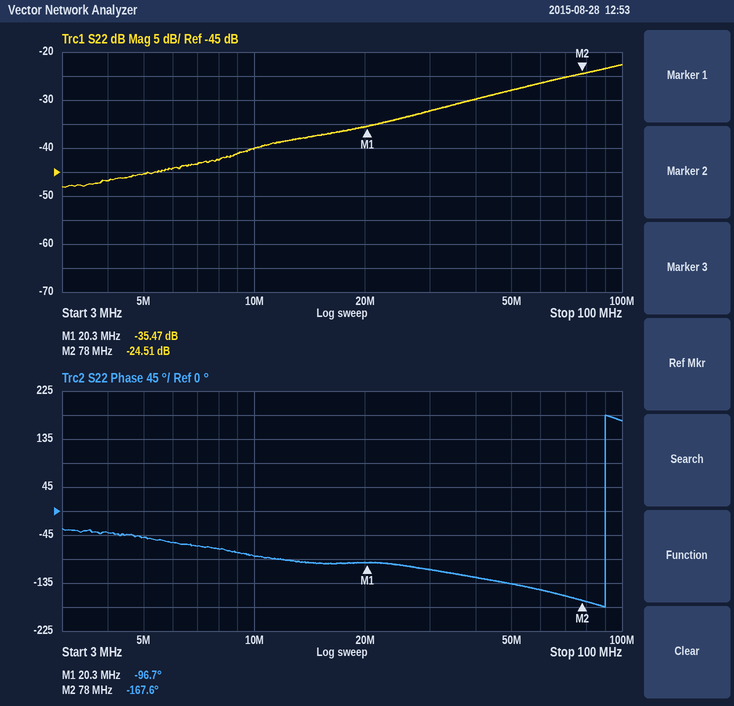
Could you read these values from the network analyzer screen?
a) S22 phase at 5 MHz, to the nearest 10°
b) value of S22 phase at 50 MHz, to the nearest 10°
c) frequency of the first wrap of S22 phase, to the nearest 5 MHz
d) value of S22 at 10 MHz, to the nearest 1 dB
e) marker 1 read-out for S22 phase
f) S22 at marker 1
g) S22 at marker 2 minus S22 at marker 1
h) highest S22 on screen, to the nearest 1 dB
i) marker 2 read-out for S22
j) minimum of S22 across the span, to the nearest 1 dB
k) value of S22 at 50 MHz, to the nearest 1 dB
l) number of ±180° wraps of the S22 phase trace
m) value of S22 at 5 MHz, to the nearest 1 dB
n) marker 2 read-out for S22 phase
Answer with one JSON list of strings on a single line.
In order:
["-50°", "-140°", "90 MHz", "-40 dB", "-96.7°", "-35.47 dB", "10.96 dB", "-23 dB", "-24.51 dB", "-48 dB", "-28 dB", "1", "-45 dB", "-167.6°"]
